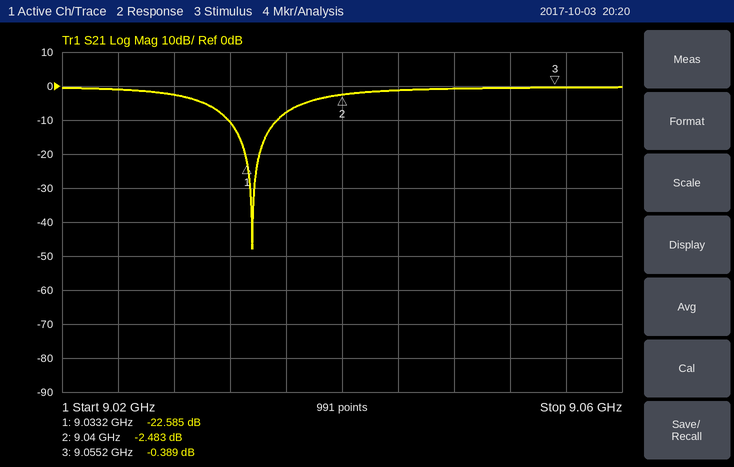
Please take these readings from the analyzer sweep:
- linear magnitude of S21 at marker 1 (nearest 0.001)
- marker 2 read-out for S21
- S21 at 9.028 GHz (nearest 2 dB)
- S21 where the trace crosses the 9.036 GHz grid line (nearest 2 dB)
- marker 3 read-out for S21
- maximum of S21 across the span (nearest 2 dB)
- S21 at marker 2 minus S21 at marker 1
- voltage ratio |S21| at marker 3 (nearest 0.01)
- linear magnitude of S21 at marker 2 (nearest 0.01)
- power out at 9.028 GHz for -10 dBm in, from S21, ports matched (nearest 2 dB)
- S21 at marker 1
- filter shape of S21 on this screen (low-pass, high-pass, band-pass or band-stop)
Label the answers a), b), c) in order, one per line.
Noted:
a) 0.074
b) -2.483 dB
c) -2 dB
d) -8 dB
e) -0.389 dB
f) 0 dB
g) 20.102 dB
h) 0.96
i) 0.75
j) -12 dBm
k) -22.585 dB
l) band-stop
